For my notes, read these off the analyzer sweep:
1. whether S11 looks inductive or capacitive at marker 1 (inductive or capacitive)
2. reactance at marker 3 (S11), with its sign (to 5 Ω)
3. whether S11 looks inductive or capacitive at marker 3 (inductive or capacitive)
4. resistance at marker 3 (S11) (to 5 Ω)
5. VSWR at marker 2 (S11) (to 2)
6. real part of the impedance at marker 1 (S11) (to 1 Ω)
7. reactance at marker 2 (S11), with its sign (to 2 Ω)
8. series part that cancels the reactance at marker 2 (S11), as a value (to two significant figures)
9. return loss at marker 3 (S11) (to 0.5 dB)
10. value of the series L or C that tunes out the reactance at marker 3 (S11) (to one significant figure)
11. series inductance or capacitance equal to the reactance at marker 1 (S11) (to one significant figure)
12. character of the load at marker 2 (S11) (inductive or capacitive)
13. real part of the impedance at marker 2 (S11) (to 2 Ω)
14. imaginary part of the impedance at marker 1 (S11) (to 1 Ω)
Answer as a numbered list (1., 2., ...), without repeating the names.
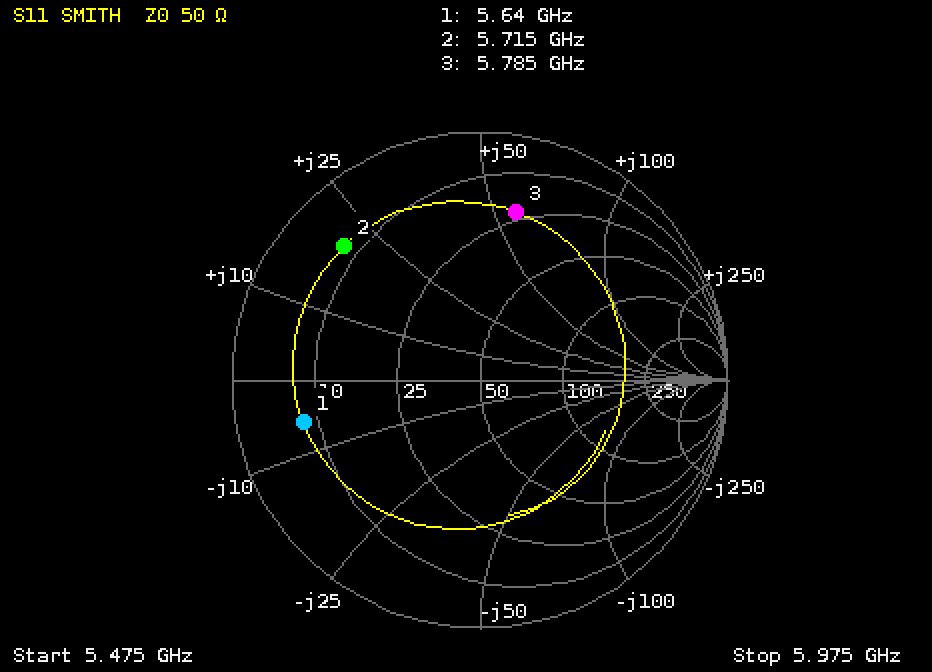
1. capacitive
2. +55 Ω
3. inductive
4. 20 Ω
5. 8
6. 8 Ω
7. +20 Ω
8. 1.4 pF
9. 3.0 dB
10. 500 fF
11. 5 pF
12. inductive
13. 8 Ω
14. -6 Ω
